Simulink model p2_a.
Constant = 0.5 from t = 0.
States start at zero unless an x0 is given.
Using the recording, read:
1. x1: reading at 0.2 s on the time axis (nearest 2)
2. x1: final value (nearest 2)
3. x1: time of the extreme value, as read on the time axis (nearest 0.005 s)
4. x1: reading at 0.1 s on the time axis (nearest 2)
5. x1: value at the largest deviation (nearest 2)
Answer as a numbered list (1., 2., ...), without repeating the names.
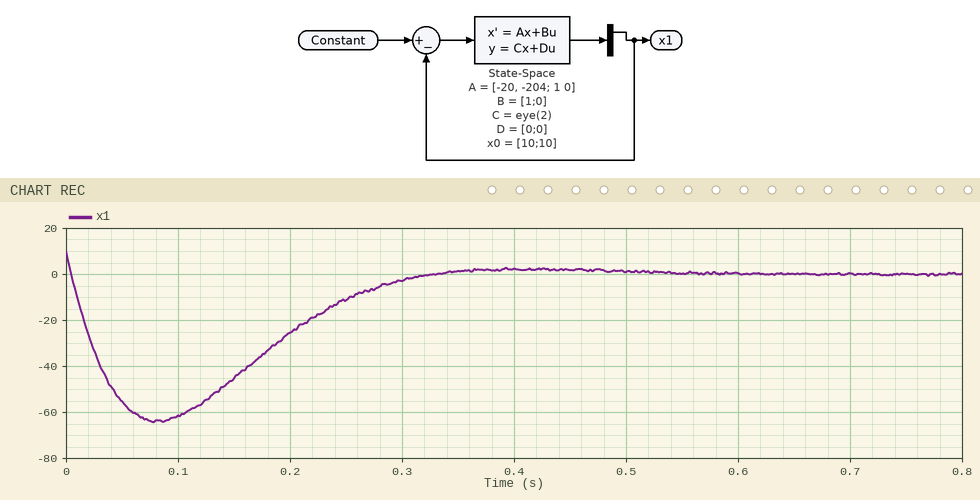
1. -26
2. 0
3. 0.080 s
4. -62
5. -64
